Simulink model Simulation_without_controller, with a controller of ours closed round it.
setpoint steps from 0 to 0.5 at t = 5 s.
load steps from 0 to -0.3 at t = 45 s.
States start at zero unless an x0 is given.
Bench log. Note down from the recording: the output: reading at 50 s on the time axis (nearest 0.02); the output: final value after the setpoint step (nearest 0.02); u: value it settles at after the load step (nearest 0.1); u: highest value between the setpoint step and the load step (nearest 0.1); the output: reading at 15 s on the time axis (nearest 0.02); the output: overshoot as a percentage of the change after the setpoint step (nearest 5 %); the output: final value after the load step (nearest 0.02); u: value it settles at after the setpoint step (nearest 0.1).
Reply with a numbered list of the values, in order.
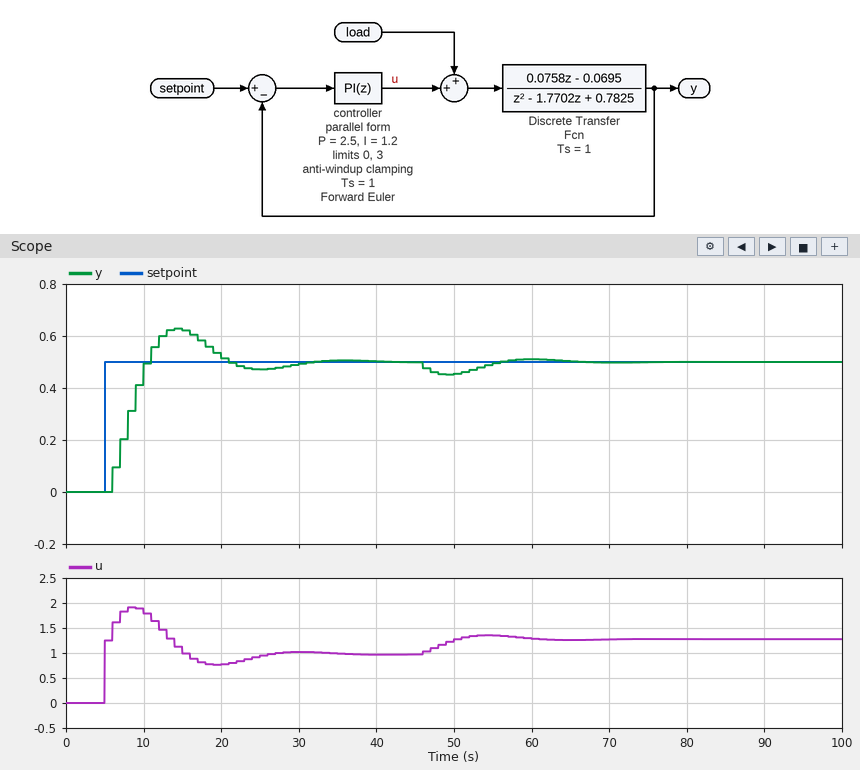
1. 0.46
2. 0.50
3. 1.3
4. 1.9
5. 0.62
6. 25 %
7. 0.50
8. 1.0
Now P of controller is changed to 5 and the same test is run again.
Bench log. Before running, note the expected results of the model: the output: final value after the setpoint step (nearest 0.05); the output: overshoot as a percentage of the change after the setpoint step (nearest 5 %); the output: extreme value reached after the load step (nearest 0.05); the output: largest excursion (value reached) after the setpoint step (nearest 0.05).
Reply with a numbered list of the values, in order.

1. 0.50
2. 10 %
3. 0.45
4. 0.55
